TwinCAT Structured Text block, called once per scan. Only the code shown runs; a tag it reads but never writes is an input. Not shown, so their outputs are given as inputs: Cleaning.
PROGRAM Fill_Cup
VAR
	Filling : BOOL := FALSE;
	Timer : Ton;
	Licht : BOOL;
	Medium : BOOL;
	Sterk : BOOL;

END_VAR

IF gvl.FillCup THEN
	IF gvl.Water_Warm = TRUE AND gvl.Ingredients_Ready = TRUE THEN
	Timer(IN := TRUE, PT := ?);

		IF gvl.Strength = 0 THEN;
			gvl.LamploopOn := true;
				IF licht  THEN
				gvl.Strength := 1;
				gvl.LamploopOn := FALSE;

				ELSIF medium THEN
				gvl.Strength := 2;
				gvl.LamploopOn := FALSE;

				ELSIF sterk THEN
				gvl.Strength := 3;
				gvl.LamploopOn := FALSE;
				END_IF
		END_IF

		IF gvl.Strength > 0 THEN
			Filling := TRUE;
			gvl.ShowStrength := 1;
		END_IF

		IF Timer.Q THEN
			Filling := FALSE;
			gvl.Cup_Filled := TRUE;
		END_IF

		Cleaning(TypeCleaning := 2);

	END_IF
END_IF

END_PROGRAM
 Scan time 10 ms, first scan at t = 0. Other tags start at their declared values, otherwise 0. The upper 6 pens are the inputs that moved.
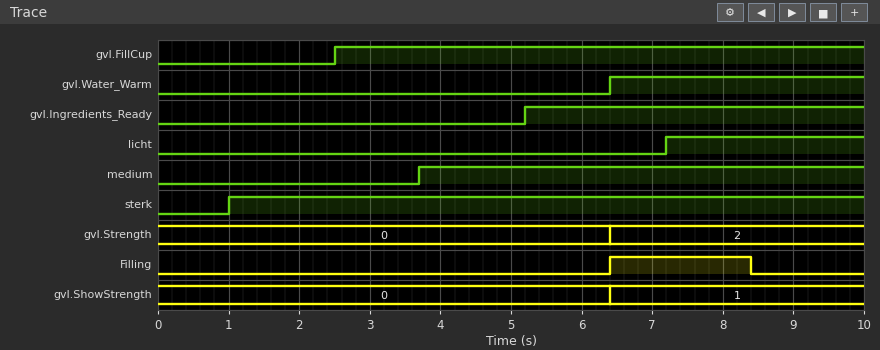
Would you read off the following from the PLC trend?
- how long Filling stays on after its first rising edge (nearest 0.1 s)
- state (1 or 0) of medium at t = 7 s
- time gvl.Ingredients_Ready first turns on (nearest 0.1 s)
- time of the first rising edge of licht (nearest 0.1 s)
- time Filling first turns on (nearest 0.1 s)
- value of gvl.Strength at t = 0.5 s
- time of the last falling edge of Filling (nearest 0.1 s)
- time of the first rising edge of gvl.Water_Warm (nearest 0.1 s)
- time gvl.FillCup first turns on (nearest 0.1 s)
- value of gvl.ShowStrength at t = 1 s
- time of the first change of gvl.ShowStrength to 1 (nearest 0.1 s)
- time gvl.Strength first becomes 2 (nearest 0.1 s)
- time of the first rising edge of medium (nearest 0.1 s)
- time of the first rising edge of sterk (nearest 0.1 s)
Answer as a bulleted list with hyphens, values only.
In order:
- 2.0 s
- 1
- 5.2 s
- 7.2 s
- 6.4 s
- 0
- 8.4 s
- 6.4 s
- 2.5 s
- 0
- 6.4 s
- 6.4 s
- 3.7 s
- 1.0 s
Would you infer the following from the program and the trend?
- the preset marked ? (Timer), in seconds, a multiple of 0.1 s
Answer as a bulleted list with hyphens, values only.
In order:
- 2.0 s
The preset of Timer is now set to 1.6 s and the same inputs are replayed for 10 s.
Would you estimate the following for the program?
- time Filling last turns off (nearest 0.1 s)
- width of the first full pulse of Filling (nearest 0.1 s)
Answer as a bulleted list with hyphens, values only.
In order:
- 8.0 s
- 1.6 s
